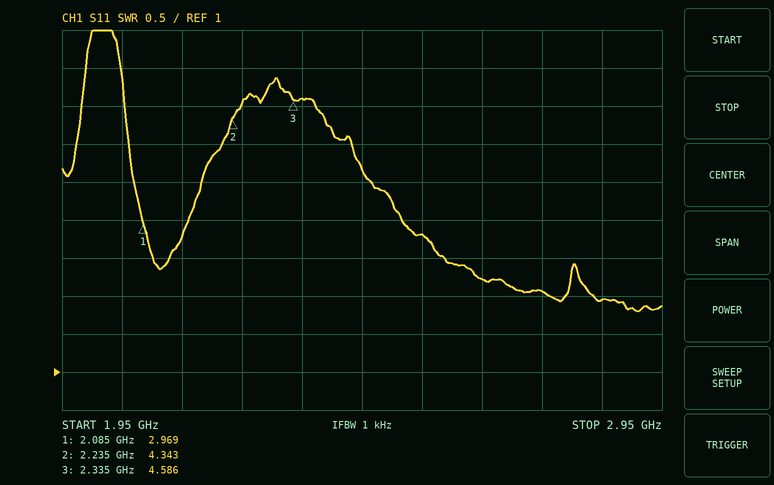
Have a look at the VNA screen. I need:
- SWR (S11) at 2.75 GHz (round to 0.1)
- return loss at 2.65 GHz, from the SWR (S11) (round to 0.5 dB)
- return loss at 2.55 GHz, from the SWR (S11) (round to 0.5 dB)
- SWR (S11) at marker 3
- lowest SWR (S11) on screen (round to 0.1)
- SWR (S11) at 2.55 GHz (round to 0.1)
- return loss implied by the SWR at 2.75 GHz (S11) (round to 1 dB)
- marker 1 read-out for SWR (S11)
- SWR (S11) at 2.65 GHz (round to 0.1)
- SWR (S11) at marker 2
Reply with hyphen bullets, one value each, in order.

- 2.1
- 8.5 dB
- 6.5 dB
- 4.586
- 1.8
- 2.8
- 9 dB
- 2.969
- 2.2
- 4.343
